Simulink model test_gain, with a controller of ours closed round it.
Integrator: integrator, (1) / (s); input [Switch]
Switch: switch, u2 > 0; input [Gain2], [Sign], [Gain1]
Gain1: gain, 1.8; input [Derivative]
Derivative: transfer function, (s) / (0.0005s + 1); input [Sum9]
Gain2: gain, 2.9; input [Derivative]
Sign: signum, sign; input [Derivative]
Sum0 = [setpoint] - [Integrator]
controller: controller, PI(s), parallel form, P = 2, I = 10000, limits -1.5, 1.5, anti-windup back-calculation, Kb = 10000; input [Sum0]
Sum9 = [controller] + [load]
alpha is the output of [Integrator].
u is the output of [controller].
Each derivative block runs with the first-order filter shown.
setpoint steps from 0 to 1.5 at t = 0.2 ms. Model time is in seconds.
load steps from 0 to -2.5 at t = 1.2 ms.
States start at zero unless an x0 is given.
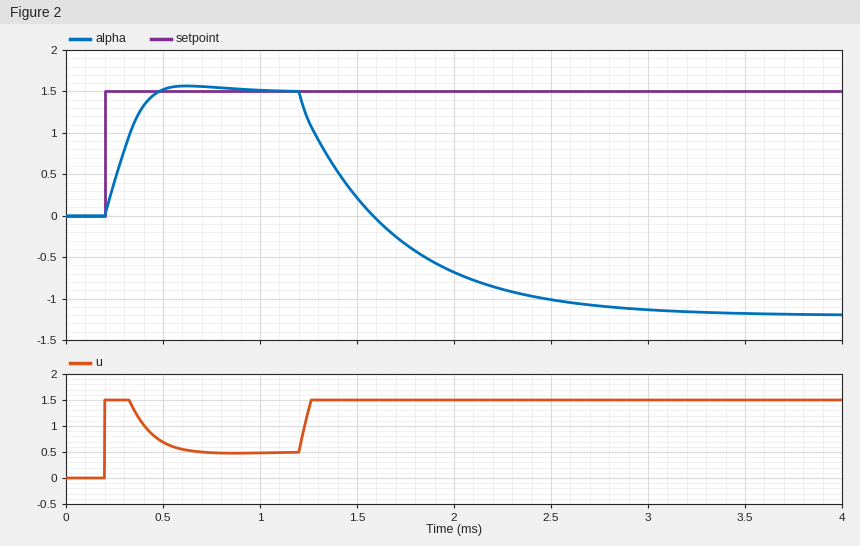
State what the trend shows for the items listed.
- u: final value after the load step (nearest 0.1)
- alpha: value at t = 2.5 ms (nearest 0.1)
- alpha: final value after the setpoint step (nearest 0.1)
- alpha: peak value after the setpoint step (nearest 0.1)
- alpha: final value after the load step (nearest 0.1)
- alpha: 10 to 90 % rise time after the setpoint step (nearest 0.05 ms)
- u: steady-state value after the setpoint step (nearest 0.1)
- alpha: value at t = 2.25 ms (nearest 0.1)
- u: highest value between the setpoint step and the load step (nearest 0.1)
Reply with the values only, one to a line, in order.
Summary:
1.5
-1.0
1.5
1.6
-1.2
0.20 ms
0.5
-0.9
1.5
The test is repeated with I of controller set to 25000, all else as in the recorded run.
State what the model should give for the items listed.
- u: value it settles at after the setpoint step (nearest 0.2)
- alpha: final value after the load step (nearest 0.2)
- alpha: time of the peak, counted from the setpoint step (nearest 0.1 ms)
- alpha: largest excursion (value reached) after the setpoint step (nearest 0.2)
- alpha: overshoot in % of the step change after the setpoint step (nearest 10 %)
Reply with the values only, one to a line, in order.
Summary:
0.4
-1.2
0.3 ms
1.8
20 %
